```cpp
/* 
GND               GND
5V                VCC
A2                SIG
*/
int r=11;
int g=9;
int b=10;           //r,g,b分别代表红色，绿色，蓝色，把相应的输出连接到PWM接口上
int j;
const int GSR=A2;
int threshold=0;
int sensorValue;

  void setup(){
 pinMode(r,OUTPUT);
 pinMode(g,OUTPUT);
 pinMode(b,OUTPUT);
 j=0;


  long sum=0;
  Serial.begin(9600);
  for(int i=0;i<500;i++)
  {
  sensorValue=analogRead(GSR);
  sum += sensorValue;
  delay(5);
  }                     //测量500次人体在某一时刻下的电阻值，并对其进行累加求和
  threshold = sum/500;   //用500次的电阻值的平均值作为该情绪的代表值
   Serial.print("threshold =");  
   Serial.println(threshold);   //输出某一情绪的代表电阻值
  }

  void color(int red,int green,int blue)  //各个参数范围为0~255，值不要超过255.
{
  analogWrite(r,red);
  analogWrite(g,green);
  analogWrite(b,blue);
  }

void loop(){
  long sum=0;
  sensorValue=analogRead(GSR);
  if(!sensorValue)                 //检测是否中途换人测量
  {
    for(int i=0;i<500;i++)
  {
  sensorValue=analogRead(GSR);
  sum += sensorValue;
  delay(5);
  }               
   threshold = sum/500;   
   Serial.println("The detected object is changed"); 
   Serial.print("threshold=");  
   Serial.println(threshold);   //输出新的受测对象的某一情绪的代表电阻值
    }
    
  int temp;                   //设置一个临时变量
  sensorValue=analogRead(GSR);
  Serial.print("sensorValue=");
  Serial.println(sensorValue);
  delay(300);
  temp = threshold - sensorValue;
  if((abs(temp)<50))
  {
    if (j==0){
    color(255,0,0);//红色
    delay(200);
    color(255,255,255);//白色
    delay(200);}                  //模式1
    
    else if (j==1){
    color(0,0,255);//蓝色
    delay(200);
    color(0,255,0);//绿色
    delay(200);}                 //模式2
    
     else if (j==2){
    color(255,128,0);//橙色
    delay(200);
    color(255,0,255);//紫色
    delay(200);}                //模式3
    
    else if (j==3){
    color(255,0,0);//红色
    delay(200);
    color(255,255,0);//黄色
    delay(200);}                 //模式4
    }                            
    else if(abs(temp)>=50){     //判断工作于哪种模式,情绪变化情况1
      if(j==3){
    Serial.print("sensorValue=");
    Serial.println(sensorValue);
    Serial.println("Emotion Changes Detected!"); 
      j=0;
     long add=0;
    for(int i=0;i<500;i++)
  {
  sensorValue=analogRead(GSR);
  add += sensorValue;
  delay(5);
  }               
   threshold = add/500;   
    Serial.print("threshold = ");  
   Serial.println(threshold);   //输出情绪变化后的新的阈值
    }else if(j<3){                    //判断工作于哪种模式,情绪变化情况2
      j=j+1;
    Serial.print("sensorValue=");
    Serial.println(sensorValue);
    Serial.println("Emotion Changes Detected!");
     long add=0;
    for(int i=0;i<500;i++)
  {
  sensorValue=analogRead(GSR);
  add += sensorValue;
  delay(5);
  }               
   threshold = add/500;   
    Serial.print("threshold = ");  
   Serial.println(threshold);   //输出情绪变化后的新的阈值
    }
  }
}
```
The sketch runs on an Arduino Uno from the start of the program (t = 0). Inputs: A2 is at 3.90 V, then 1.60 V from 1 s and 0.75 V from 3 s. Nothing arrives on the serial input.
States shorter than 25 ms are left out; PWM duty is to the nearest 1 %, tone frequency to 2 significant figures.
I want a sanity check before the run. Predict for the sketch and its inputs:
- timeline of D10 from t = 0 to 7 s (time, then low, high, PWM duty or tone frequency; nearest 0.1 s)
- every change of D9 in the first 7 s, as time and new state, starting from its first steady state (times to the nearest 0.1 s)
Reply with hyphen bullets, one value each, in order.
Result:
- 0 s low; 5.7 s high; 5.9 s low; 6.4 s high; 6.6 s low
- 0 s low; 5.9 s high; 6.4 s low; 6.6 s high
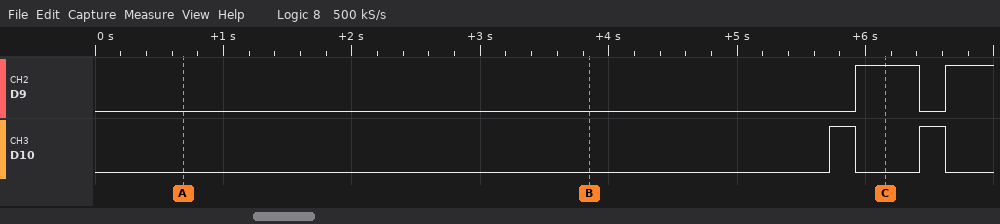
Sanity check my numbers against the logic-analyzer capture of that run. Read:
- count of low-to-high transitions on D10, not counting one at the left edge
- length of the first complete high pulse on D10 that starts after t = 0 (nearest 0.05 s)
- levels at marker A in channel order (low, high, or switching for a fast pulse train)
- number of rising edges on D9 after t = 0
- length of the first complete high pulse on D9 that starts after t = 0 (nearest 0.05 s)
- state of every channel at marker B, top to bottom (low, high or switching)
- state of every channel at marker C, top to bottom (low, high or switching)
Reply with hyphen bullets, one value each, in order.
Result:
- 2
- 0.20 s
- D9 low, D10 low
- 2
- 0.50 s
- D9 low, D10 low
- D9 high, D10 low
